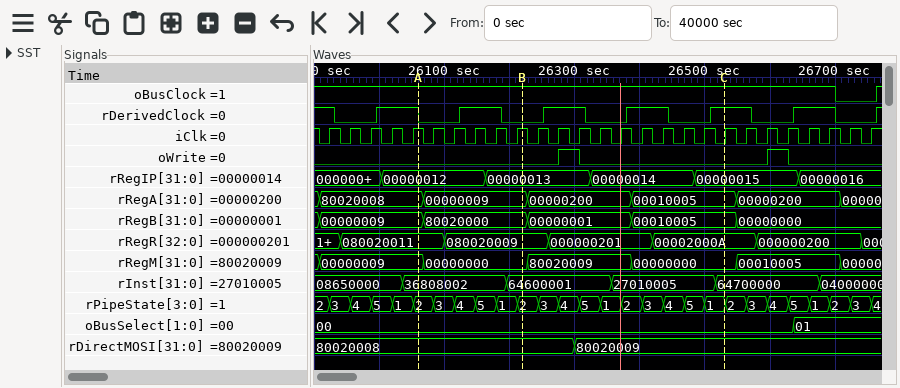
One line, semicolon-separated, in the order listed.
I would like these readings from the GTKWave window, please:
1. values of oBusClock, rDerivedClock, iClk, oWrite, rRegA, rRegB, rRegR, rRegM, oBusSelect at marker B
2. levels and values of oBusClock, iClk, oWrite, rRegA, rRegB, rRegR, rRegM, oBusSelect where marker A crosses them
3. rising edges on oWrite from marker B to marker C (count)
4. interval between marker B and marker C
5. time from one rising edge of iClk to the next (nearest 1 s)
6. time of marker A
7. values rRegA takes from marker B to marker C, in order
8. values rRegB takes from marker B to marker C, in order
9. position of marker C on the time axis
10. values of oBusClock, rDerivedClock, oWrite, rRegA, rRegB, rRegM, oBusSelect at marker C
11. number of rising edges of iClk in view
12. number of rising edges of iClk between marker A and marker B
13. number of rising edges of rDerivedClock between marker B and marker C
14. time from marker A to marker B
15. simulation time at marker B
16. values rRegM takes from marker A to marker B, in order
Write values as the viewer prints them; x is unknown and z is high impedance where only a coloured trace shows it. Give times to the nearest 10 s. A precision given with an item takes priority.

oBusClock=1, rDerivedClock=0, iClk=1, oWrite=0, rRegA=00000009, rRegB=80020000, rRegR=080020009, rRegM=00000000, oBusSelect=00; oBusClock=1, iClk=1, oWrite=0, rRegA=80020008, rRegB=00000009, rRegR=080020011, rRegM=00000009, oBusSelect=00; 1; 310 s; 32 s; 26060 s; 00000009, 00000200, 00010005; 80020000, 00000001, 00010005; 26530 s; oBusClock=1, rDerivedClock=1, oWrite=0, rRegA=00010005, rRegB=00010005, rRegM=00000000, oBusSelect=00; 27; 5; 3; 160 s; 26220 s; 00000009, 00000000
